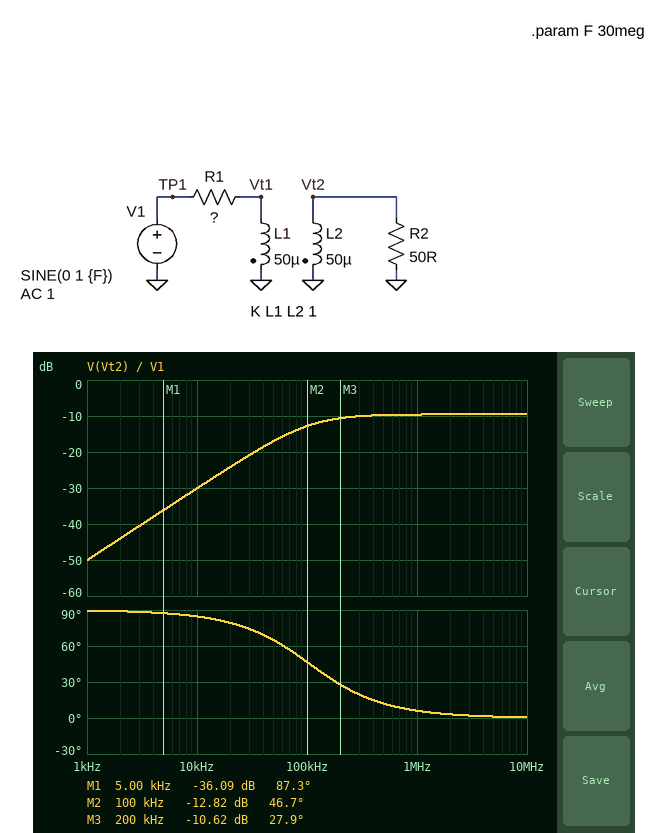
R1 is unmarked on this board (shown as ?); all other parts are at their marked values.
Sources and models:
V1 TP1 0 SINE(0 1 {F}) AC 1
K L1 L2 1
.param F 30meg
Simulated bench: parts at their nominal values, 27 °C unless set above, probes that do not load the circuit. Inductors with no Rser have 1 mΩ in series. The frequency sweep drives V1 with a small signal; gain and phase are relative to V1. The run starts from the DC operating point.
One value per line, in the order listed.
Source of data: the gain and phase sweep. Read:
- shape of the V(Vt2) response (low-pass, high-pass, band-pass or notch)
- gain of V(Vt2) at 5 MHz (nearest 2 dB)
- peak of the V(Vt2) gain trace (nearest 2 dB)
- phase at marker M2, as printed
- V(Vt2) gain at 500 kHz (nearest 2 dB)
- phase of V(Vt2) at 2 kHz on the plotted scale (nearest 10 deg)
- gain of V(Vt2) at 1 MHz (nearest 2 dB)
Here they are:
high-pass
-10 dB
-10 dB
46.7 deg
-10 dB
90 deg
-10 dB
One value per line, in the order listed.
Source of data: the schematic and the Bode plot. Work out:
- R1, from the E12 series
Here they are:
100 Ω
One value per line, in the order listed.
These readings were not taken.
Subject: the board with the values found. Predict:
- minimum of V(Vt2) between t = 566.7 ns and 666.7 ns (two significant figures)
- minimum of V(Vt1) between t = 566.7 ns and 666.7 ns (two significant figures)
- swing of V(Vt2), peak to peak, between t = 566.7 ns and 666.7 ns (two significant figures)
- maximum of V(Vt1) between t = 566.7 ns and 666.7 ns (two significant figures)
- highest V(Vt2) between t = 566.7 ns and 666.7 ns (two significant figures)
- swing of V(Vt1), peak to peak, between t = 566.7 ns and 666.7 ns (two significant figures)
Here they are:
-330 mV
-330 mV
670 mV
330 mV
330 mV
670 mV
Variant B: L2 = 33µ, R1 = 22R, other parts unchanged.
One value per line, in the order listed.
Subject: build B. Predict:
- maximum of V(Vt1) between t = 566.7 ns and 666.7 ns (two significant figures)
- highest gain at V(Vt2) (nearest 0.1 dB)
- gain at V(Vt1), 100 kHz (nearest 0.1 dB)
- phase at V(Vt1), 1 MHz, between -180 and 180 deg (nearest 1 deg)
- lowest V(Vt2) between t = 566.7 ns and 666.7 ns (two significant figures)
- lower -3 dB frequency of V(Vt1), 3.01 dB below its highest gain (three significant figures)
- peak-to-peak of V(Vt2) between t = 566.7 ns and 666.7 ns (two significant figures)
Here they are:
770 mV
-4.0 dB
-3.3 dB
3 deg
-630 mV
54.3 kHz
1.3 V
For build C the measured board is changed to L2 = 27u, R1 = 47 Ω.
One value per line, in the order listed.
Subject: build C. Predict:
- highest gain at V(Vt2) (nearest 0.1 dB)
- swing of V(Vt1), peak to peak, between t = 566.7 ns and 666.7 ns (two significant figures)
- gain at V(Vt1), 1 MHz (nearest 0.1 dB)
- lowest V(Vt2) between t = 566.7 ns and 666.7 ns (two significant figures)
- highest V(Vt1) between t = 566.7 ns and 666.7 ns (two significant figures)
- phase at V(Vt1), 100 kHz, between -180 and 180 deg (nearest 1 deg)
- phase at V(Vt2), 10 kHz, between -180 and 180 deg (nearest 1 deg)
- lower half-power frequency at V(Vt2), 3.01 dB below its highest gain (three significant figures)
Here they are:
-6.2 dB
1.3 V
-3.6 dB
-490 mV
660 mV
45 deg
84 deg
99.2 kHz
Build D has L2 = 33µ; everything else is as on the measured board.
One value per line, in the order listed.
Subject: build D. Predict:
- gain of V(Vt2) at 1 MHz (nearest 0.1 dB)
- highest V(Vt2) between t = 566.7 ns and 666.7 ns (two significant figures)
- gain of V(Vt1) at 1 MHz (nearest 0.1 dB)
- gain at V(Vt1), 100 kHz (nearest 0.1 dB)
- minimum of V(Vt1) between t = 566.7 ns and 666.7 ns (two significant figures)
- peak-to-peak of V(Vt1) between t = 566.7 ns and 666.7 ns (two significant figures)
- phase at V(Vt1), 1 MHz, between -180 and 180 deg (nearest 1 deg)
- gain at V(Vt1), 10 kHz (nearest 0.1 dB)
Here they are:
-9.2 dB
350 mV
-7.4 dB
-11.9 dB
-430 mV
860 mV
8 deg
-30.1 dB
